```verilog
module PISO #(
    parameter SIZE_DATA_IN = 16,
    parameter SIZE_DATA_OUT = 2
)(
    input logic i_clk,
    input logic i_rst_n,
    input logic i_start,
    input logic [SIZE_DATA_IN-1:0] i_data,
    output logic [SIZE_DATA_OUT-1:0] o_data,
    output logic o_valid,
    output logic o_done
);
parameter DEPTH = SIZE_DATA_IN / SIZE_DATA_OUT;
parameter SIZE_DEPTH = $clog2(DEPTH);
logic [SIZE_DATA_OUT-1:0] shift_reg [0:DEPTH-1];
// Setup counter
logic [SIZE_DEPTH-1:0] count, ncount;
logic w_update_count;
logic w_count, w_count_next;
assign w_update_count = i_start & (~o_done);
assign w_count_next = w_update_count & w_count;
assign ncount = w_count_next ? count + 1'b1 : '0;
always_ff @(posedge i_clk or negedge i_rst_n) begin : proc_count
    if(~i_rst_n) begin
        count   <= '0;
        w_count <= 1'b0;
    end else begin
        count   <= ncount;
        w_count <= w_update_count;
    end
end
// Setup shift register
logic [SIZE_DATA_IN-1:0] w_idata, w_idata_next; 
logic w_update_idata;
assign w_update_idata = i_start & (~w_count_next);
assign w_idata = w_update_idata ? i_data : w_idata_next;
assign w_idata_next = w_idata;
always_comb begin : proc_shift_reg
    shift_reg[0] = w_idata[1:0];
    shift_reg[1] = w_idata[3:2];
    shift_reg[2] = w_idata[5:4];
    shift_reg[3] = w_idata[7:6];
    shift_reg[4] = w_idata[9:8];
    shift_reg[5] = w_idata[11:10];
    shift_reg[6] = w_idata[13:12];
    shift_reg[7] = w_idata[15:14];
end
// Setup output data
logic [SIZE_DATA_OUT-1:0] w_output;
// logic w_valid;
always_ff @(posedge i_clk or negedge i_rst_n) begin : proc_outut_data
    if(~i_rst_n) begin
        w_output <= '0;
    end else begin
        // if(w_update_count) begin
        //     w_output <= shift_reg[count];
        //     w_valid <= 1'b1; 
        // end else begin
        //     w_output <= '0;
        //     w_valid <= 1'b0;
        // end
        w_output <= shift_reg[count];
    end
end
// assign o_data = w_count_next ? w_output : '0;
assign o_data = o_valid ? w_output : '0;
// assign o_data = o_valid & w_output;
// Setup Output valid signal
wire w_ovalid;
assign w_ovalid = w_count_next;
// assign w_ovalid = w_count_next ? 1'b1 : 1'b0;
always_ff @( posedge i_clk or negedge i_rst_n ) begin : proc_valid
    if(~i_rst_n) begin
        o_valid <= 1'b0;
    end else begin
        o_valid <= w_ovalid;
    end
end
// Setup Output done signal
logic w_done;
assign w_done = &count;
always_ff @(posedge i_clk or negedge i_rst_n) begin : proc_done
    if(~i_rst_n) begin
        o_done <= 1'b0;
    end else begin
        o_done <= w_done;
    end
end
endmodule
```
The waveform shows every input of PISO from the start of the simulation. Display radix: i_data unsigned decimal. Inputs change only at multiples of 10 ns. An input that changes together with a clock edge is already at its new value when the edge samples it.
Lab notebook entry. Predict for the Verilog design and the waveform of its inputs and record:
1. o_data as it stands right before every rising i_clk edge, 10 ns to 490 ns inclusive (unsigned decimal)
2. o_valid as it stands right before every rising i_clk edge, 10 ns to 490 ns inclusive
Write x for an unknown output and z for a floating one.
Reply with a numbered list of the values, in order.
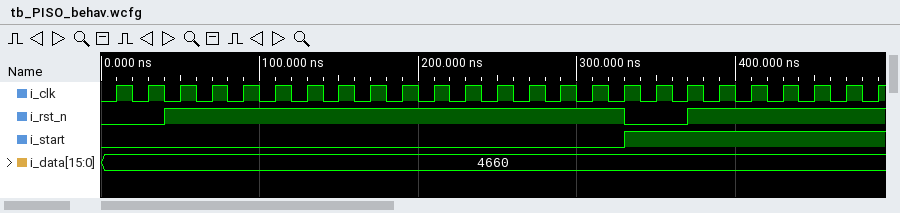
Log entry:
1. 0, 0, 0, 0, 0, 0, 0, 0, 0, 0, 0, 0, 0, 0, 0, 0, 0, 0, 0, 0, 0, 1, 3, 0, 2
2. 0 0 0 0 0 0 0 0 0 0 0 0 0 0 0 0 0 0 0 0 1 1 1 1 1
